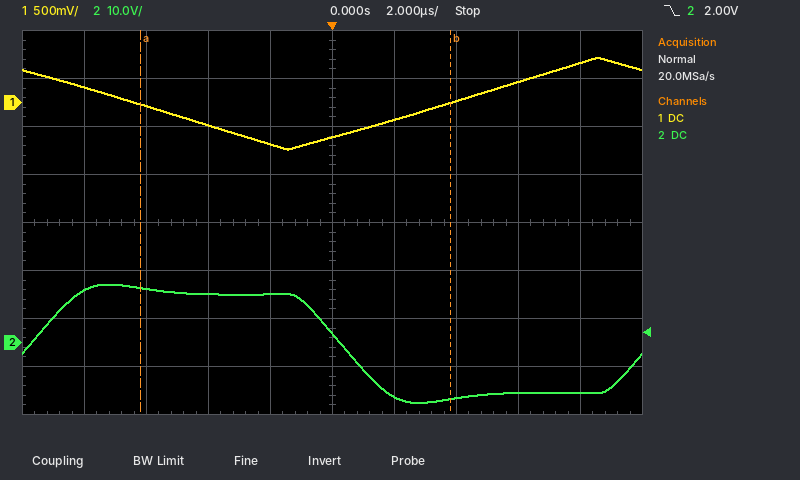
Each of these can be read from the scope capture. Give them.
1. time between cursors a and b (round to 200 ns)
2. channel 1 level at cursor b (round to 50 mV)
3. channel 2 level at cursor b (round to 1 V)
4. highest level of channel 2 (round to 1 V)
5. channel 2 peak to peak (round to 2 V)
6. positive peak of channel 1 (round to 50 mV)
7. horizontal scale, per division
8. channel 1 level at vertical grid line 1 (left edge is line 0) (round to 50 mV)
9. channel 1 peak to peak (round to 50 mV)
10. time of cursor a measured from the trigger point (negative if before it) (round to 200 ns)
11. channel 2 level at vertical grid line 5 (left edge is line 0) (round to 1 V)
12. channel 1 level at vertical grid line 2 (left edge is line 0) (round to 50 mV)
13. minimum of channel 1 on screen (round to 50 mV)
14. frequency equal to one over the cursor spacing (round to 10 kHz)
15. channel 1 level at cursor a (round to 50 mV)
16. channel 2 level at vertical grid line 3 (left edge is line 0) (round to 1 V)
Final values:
10.0 µs
0 mV
-12 V
12 V
24 V
450 mV
2 µs
150 mV
950 mV
-6.2 µs
2 V
-50 mV
-500 mV
100 kHz
0 mV
10 V
